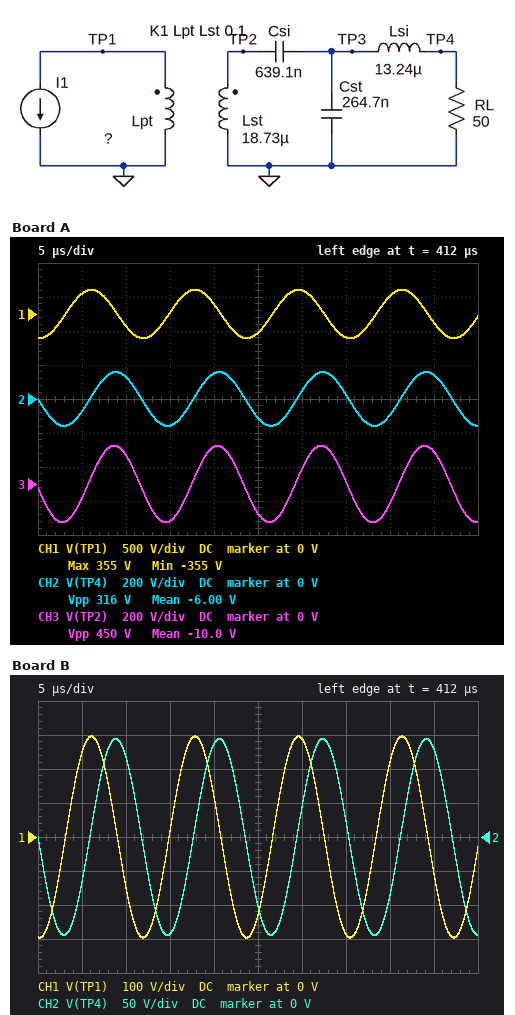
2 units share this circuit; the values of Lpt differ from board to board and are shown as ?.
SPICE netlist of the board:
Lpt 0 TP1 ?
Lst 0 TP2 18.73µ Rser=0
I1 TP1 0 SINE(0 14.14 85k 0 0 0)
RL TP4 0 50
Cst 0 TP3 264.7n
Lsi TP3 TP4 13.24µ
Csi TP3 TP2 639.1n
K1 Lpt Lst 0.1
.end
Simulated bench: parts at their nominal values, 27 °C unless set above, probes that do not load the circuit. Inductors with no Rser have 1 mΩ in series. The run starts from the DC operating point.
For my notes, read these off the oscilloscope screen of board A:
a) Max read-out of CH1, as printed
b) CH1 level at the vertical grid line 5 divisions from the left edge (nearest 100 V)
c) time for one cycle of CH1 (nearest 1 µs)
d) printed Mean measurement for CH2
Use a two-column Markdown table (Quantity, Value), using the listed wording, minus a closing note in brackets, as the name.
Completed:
| Quantity | Value |
|---|---|
| Max read-out of CH1, as printed | 355 V |
| CH1 level at the vertical grid line 5 divisions from the left edge | -300 V |
| time for one cycle of CH1 | 12 µs |
| printed Mean measurement for CH2 | -6.00 V |
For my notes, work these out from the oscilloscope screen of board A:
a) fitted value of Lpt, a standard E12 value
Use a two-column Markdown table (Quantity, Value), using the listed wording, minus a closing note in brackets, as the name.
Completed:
| Quantity | Value |
|---|---|
| fitted value of Lpt, a standard E12 value | 47 µH |
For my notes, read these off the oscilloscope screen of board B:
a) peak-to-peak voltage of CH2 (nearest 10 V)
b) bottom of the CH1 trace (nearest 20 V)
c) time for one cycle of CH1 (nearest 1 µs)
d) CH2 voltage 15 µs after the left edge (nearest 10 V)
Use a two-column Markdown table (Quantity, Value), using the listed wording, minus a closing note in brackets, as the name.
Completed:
| Quantity | Value |
|---|---|
| peak-to-peak voltage of CH2 | 290 V |
| bottom of the CH1 trace | -300 V |
| time for one cycle of CH1 | 12 µs |
| CH2 voltage 15 µs after the left edge | -140 V |
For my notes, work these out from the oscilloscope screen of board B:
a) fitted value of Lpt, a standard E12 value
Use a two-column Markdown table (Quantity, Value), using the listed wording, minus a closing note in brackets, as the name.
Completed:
| Quantity | Value |
|---|---|
| fitted value of Lpt, a standard E12 value | 39 µH |
